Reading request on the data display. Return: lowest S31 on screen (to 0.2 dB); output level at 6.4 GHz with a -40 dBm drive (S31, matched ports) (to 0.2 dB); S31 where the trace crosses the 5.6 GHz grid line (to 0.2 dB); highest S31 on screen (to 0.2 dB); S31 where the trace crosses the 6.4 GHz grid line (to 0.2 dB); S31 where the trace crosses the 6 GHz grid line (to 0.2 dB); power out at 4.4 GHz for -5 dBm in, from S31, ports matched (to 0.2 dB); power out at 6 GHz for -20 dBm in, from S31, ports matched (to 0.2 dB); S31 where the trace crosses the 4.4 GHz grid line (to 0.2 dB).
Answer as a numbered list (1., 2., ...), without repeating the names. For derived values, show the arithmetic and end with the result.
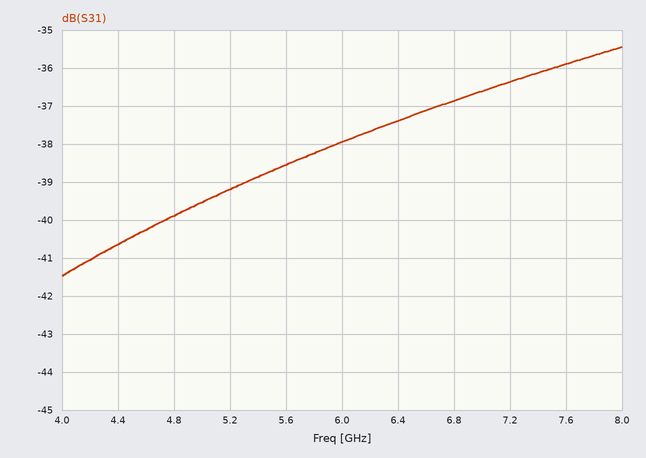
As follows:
1. -41.4 dB
2. -40 dBm + (-37.4 dB) = -77.4 dBm
3. -38.6 dB
4. -35.4 dB
5. -37.4 dB
6. -38.0 dB
7. -5 dBm + (-40.6 dB) = -45.6 dBm
8. -20 dBm + (-38.0 dB) = -58.0 dBm
9. -40.6 dB
